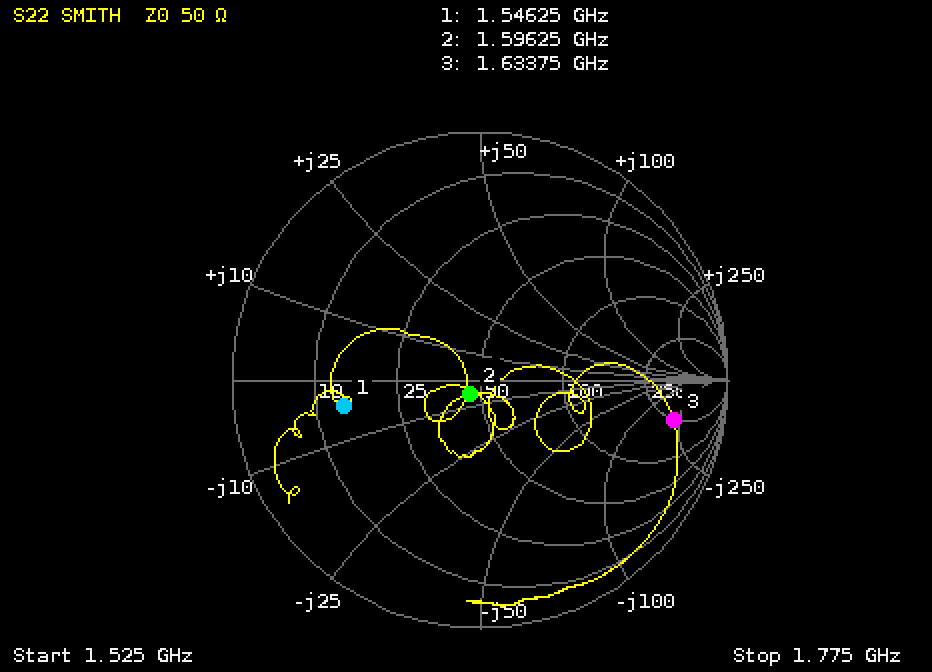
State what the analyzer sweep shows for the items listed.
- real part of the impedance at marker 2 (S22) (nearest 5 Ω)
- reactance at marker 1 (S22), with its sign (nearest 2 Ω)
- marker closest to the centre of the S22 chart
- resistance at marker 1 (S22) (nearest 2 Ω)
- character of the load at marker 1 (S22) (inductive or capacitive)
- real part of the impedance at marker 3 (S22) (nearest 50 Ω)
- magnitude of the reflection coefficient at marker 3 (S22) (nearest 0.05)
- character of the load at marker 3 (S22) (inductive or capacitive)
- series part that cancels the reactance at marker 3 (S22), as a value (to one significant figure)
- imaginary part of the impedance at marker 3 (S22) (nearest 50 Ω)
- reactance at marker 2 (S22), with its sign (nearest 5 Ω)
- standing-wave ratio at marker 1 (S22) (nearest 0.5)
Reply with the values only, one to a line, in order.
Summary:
45 Ω
-4 Ω
marker 2
14 Ω
capacitive
250 Ω
0.80
capacitive
20 nH
-200 Ω
-5 Ω
3.5
